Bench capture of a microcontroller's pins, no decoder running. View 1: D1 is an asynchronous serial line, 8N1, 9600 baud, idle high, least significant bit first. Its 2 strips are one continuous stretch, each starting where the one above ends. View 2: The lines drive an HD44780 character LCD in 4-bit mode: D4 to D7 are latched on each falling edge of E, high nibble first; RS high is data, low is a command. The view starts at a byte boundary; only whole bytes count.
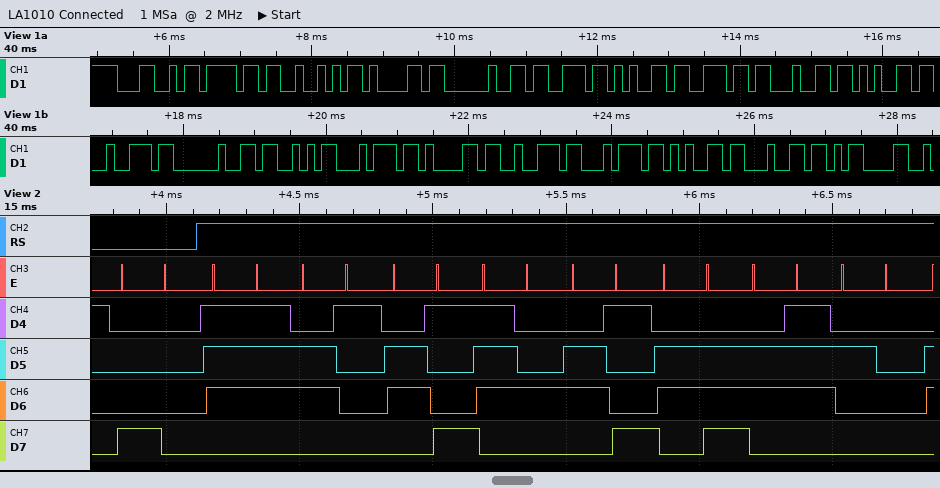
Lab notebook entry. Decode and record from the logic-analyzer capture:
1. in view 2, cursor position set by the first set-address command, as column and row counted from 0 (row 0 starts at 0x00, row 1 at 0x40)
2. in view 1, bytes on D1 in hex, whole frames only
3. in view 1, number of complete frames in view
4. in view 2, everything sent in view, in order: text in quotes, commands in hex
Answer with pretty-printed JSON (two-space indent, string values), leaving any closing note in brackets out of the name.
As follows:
{
  "in view 2, cursor position set by the first set-address command, as column and row counted from 0": "column 0, row 0",
  "in view 1, bytes on D1 in hex, whole frames only": "0x4C 0x6F 0x52 0x61 0x20 0x73 0x65 0x6E 0x64 0x65 0x72 0x20 0x53 0x74 0x61 0x72 0x74 0x65 0x64 0x0D",
  "in view 1, number of complete frames in view": "20",
  "in view 2, everything sent in view, in order: text in quotes, commands in hex": "0x80 \"waiting \""
}
